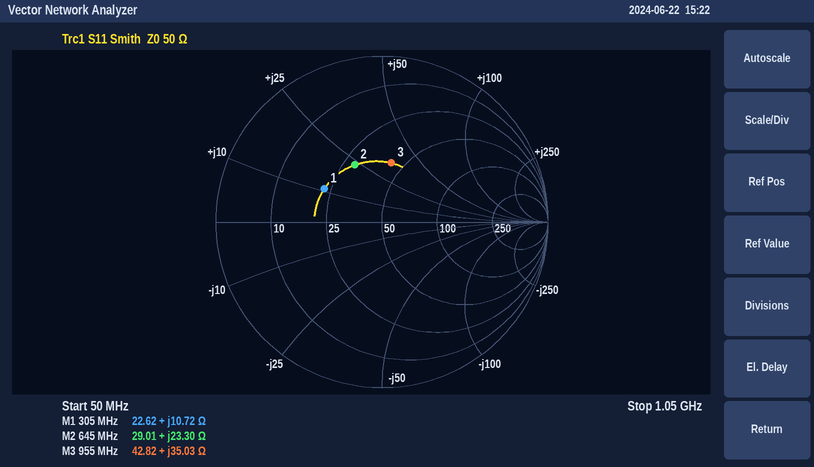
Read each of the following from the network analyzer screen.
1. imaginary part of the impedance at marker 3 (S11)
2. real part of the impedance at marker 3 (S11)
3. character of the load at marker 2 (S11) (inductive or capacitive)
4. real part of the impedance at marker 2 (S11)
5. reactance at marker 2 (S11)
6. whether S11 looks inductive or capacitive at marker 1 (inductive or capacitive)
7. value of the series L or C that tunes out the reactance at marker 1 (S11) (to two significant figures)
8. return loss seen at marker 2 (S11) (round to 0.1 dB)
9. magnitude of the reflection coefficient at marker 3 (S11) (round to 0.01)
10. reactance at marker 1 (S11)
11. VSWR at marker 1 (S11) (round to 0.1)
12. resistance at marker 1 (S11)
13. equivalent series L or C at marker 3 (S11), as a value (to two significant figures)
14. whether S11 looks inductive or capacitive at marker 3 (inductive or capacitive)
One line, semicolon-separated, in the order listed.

+35.03 Ω; 42.82 Ω; inductive; 29.01 Ω; +23.30 Ω; inductive; 49 pF; 8.4 dB; 0.36; +10.72 Ω; 2.3; 22.62 Ω; 5.8 nH; inductive
